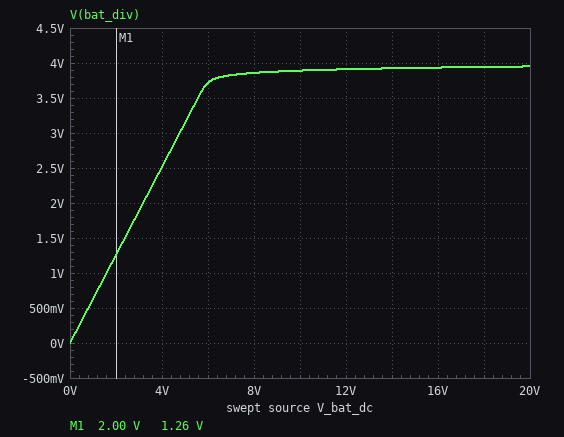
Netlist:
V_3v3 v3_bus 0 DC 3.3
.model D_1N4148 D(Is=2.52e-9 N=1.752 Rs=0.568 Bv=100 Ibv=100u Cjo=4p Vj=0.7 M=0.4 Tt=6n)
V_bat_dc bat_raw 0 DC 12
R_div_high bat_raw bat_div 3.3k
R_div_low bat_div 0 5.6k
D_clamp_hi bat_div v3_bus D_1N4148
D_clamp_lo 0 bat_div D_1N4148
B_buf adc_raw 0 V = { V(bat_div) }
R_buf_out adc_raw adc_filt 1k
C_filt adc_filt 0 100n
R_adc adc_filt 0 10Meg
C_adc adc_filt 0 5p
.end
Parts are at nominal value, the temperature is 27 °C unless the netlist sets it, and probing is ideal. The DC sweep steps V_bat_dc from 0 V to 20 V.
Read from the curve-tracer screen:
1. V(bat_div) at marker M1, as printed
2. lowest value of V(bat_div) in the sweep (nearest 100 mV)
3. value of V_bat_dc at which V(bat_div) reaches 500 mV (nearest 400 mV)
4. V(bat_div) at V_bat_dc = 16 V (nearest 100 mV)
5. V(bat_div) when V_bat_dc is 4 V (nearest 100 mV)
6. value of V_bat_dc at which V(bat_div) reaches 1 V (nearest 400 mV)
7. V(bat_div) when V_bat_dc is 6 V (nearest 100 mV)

1.26 V
0 V
800 mV
3.9 V
2.5 V
1.6 V
3.7 V
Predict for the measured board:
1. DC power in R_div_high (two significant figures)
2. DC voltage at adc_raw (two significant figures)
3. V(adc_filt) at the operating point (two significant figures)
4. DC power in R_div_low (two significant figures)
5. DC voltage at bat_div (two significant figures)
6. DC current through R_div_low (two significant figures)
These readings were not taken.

20 mW
3.9 V
3.9 V
2.7 mW
3.9 V
700 µA
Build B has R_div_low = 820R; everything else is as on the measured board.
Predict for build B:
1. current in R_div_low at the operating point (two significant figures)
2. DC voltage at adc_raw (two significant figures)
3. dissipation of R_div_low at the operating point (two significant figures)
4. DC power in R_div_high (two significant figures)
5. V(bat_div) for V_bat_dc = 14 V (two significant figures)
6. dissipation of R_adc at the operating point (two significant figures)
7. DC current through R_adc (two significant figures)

2.9 mA
2.4 V
7.0 mW
28 mW
2.8 V
570 nW
240 nA
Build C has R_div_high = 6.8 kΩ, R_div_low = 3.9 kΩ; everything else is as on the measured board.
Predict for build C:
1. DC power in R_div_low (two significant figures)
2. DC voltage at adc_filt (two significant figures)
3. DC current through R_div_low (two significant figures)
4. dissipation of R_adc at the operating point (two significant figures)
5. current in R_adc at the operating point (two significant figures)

3.7 mW
3.8 V
980 µA
1.5 µW
380 nA
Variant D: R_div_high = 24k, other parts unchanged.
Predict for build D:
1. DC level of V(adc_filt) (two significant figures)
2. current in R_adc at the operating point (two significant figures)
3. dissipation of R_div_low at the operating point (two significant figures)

2.3 V
230 nA
920 µW
